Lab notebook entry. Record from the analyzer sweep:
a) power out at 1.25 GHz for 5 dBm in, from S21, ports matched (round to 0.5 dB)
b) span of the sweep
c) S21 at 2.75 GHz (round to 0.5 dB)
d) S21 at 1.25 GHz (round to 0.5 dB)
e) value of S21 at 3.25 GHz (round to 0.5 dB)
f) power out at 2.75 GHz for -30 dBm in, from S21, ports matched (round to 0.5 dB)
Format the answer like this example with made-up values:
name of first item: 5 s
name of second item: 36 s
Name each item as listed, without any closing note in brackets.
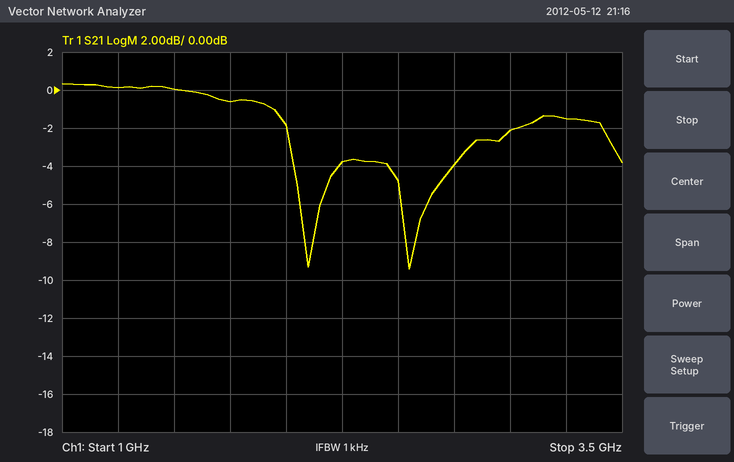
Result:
power out at 1.25 GHz for 5 dBm in, from S21, ports matched: 5.0 dBm
span of the sweep: 2.5 GHz
S21 at 2.75 GHz: -4.0 dB
S21 at 1.25 GHz: 0.0 dB
value of S21 at 3.25 GHz: -1.5 dB
power out at 2.75 GHz for -30 dBm in, from S21, ports matched: -34.0 dBm
